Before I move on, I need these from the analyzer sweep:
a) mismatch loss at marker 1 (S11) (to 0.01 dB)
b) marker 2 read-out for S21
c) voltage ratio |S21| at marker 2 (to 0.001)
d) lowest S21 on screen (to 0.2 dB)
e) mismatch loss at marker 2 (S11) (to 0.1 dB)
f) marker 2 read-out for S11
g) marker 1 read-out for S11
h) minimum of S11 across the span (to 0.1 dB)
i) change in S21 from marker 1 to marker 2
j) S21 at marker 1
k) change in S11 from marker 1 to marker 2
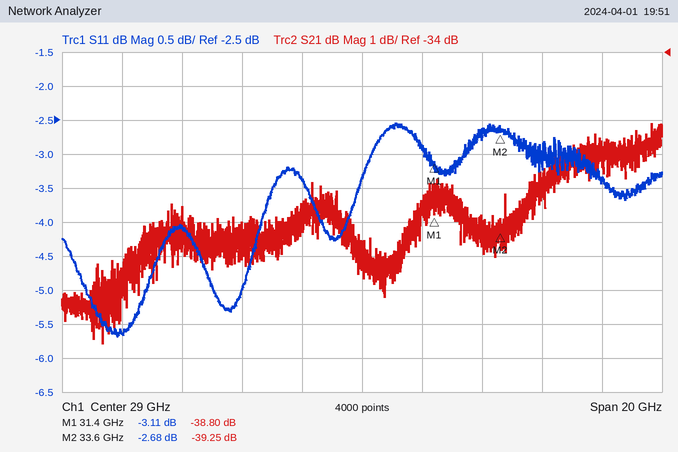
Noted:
2.91 dB
-39.25 dB
0.011
-42.6 dB
3.4 dB
-2.68 dB
-3.11 dB
-5.7 dB
-0.45 dB
-38.80 dB
0.43 dB
